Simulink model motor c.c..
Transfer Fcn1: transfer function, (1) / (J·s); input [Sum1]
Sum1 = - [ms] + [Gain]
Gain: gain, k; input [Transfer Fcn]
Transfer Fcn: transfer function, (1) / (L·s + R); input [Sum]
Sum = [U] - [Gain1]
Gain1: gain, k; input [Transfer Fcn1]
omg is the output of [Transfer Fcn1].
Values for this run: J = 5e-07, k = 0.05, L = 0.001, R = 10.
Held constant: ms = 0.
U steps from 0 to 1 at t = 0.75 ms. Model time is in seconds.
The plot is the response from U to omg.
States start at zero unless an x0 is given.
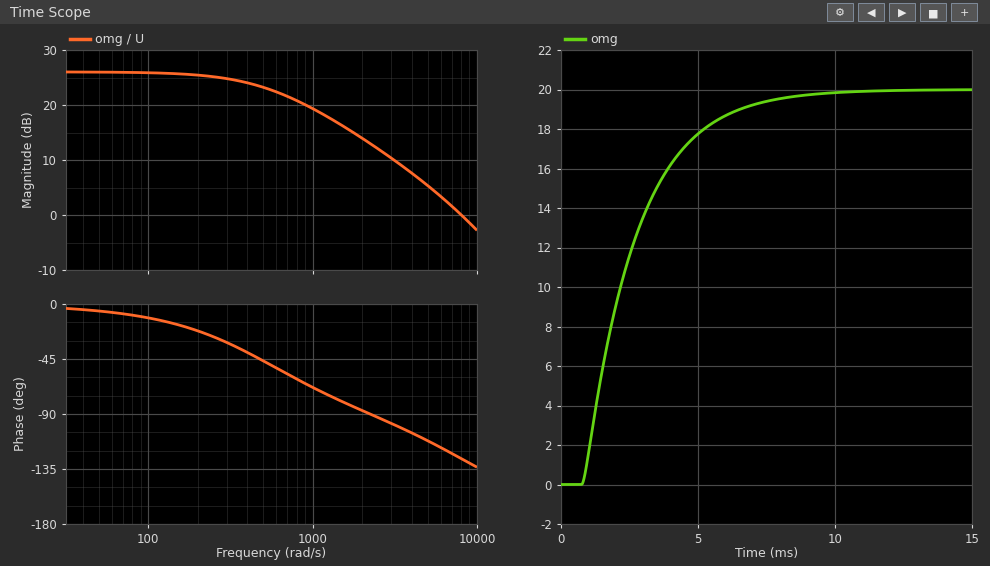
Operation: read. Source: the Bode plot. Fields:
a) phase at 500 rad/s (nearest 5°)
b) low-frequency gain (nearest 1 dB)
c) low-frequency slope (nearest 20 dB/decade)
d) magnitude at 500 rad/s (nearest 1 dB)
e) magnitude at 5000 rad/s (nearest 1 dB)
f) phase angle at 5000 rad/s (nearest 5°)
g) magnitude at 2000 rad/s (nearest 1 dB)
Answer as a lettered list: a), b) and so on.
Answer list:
a) -45°
b) 26 dB
c) 0 dB/decade
d) 23 dB
e) 5 dB
f) -110°
g) 14 dB
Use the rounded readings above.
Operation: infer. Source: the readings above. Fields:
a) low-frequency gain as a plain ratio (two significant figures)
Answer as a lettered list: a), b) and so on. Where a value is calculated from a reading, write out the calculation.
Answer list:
a) 10^(26 / 20) = 20
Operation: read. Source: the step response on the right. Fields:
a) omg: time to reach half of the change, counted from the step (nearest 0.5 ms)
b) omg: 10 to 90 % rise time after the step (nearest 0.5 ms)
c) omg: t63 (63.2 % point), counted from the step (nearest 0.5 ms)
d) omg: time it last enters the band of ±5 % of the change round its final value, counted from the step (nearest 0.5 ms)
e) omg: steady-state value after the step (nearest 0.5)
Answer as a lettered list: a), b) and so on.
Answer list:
a) 1.5 ms
b) 4.0 ms
c) 2.0 ms
d) 6.0 ms
e) 20.0
